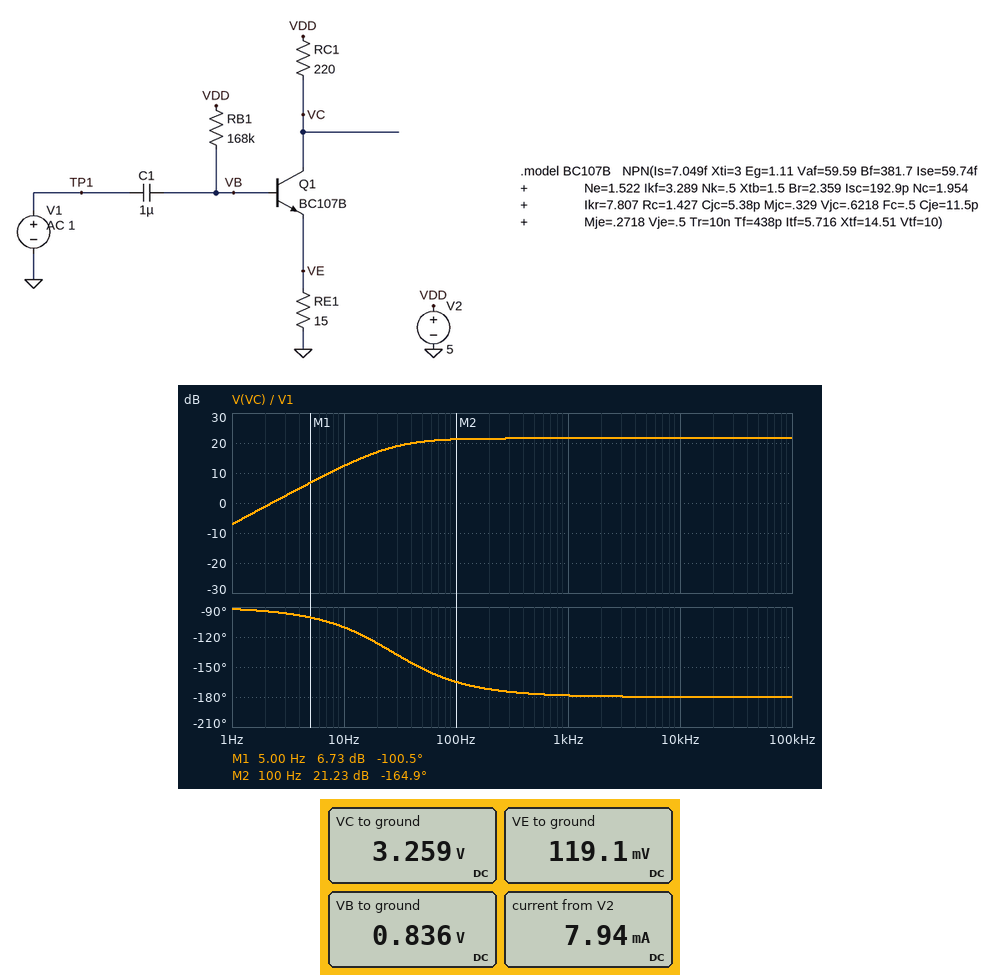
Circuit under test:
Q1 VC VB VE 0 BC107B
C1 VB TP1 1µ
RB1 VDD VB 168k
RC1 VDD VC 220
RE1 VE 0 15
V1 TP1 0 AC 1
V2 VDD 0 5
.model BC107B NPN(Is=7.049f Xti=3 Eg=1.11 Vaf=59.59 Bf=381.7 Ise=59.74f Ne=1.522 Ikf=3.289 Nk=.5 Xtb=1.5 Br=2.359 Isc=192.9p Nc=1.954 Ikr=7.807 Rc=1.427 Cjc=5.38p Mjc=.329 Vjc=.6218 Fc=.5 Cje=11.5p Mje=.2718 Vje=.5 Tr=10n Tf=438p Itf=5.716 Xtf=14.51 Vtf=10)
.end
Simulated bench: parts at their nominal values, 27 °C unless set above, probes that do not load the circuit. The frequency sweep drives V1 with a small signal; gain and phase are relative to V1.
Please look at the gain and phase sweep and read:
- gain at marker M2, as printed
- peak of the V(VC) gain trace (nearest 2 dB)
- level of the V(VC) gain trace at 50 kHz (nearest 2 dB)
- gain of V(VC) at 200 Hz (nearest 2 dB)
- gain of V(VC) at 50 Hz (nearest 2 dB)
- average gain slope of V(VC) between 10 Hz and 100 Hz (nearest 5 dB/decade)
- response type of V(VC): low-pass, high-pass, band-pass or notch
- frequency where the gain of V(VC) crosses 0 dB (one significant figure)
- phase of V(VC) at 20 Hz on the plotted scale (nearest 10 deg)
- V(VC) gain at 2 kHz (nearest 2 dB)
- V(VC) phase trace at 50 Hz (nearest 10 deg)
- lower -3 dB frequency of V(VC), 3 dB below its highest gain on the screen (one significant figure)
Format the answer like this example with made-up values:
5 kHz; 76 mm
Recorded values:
21.23 dB; 22 dB; 22 dB; 22 dB; 20 dB; 10 dB/decade; high-pass; 2 Hz; -130 deg; 22 dB; -150 deg; 30 Hz
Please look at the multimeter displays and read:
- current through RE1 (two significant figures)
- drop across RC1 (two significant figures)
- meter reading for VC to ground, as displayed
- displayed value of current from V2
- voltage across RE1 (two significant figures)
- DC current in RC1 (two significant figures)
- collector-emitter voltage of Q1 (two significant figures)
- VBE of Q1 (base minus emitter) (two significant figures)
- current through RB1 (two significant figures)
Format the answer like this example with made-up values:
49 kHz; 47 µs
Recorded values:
7.9 mA; 1.7 V; 3.259 V; 7.94 mA; 120 mV; 7.9 mA; 3.1 V; 720 mV; 25 µA
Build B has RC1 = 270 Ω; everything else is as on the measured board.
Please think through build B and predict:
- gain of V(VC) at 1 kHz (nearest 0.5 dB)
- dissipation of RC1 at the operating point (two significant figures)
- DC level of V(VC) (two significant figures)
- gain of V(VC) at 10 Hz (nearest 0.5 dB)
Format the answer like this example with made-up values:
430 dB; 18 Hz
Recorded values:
23.5 dB; 17 mW; 2.9 V; 14.0 dB
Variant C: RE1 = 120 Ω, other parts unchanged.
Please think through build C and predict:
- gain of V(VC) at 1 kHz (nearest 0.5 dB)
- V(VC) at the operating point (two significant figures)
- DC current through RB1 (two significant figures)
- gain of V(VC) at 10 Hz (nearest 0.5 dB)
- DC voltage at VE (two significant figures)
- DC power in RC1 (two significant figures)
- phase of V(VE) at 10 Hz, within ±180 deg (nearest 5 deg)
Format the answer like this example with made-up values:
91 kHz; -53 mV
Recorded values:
5.0 dB; 3.6 V; 21 µA; 4.0 dB; 790 mV; 9.4 mW; 25 deg
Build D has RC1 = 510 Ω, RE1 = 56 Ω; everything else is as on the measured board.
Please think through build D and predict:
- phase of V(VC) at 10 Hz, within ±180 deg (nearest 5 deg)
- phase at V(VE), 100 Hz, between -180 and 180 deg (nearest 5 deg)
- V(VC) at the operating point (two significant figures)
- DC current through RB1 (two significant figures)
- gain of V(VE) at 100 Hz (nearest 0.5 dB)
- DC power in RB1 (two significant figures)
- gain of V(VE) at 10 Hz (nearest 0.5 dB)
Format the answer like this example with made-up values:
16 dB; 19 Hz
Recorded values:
-135 deg; 5 deg; 1.4 V; 23 µA; -0.5 dB; 90 µW; -3.5 dB
